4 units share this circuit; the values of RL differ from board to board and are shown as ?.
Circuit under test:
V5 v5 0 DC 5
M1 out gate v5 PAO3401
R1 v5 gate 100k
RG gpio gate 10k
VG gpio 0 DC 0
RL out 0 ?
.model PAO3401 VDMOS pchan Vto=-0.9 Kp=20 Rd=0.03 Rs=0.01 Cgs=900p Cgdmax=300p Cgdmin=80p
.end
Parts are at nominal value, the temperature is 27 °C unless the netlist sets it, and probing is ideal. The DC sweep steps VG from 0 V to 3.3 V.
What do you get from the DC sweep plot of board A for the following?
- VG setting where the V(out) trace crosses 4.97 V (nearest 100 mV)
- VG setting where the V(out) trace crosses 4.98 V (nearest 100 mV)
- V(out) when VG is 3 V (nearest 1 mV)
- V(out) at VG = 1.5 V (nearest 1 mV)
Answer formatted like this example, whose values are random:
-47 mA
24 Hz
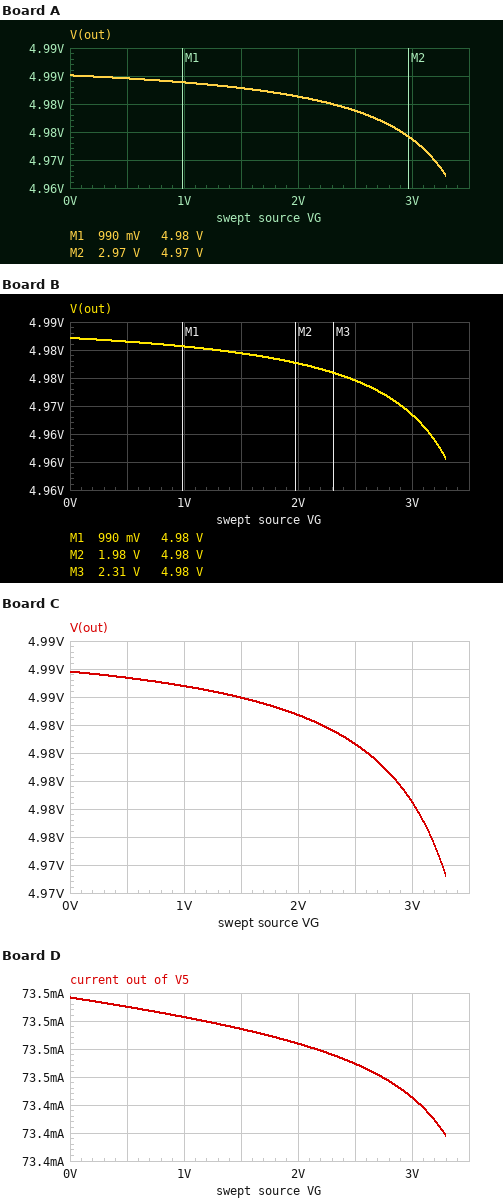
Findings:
3.2 V
2.9 V
4.974 V
4.983 V
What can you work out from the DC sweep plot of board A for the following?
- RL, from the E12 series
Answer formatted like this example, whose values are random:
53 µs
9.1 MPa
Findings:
18 Ω
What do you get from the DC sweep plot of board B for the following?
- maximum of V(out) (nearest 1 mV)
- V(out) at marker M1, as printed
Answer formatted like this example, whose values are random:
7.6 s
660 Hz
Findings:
4.982 V
4.98 V
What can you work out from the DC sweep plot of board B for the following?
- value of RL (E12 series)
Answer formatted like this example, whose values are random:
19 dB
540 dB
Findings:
15 Ω
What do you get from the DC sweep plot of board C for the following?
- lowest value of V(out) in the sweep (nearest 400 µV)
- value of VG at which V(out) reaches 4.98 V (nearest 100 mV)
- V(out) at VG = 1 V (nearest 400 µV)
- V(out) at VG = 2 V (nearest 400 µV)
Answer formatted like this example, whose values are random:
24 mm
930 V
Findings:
4.9732 V
3.2 V
4.9868 V
4.9848 V
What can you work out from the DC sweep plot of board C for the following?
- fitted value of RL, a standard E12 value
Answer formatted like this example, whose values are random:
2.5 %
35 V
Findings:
22 Ω
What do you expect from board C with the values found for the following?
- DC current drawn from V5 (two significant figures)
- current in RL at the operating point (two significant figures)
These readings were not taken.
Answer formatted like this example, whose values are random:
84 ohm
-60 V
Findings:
230 mA
230 mA
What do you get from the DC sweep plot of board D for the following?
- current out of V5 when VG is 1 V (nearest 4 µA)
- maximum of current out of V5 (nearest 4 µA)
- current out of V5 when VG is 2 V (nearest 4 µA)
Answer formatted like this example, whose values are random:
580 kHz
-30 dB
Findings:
73.504 mA
73.516 mA
73.484 mA
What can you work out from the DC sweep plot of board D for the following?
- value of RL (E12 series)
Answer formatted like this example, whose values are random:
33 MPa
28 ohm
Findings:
68 Ω
